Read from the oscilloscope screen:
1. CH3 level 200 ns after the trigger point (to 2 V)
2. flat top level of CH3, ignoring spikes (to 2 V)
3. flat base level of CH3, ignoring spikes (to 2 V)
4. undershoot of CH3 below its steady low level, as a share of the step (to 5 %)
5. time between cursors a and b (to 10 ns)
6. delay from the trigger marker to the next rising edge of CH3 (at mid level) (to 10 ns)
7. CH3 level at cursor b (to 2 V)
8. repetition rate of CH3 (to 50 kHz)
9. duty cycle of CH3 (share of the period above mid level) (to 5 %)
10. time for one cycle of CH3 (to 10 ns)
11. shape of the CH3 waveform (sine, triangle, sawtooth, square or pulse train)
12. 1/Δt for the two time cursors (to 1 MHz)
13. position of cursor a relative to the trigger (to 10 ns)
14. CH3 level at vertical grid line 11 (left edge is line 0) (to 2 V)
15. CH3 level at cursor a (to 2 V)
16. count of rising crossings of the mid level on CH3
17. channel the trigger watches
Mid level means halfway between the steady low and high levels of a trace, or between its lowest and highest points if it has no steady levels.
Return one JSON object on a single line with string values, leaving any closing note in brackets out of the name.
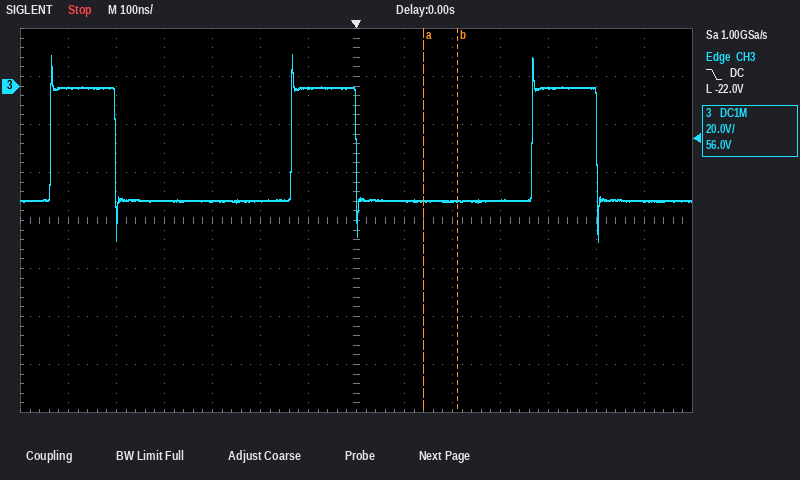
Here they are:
{"CH3 level 200 ns after the trigger point": "-48 V", "flat top level of CH3, ignoring spikes": "0 V", "flat base level of CH3, ignoring spikes": "-48 V", "undershoot of CH3 below its steady low level, as a share of the step": "35 %", "time between cursors a and b": "70 ns", "delay from the trigger marker to the next rising edge of CH3 (at mid level)": "370 ns", "CH3 level at cursor b": "-48 V", "repetition rate of CH3": "2.00 MHz", "duty cycle of CH3 (share of the period above mid level)": "25 %", "time for one cycle of CH3": "500 ns", "shape of the CH3 waveform": "pulse train", "1/Δt for the two time cursors": "14 MHz", "position of cursor a relative to the trigger": "+140 ns", "CH3 level at vertical grid line 11 (left edge is line 0)": "0 V", "CH3 level at cursor a": "-48 V", "count of rising crossings of the mid level on CH3": "3", "channel the trigger watches": "CH3"}
